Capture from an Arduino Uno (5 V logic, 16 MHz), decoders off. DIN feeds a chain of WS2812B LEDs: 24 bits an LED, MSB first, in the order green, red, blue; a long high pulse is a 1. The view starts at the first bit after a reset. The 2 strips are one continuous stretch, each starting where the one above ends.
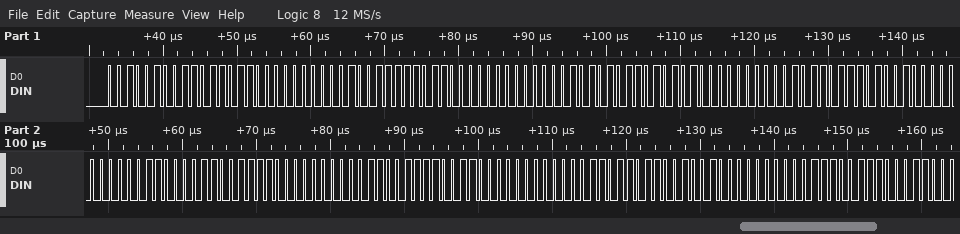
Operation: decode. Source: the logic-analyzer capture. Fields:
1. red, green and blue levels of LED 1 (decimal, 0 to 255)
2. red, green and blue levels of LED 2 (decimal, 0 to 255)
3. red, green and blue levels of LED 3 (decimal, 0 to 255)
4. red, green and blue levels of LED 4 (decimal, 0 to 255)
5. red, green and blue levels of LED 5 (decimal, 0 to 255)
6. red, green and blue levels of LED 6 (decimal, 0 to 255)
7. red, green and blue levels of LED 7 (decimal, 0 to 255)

219, 36, 0
216, 39, 0
213, 42, 0
210, 45, 0
207, 48, 0
204, 51, 0
201, 54, 0
